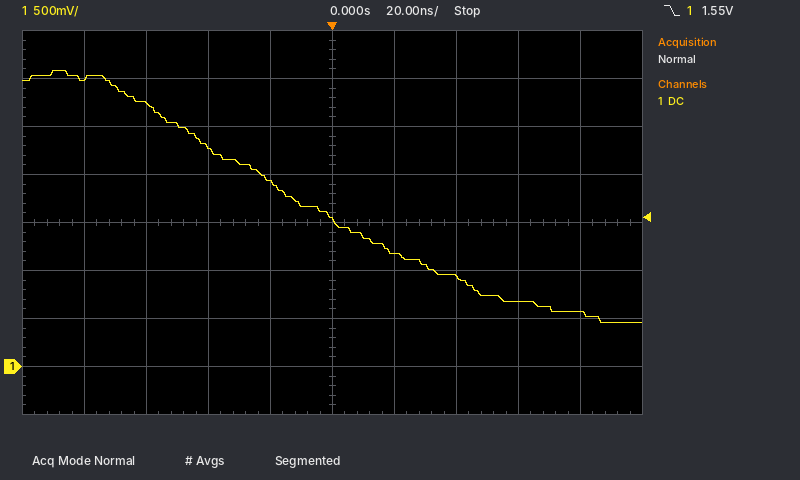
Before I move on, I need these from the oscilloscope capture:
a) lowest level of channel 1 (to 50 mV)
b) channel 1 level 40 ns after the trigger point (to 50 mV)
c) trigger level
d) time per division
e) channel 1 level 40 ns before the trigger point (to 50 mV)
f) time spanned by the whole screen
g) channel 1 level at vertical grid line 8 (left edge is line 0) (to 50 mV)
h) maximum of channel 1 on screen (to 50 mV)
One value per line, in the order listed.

450 mV
950 mV
1.55 V
20 ns
2.30 V
200 ns
700 mV
3.10 V
